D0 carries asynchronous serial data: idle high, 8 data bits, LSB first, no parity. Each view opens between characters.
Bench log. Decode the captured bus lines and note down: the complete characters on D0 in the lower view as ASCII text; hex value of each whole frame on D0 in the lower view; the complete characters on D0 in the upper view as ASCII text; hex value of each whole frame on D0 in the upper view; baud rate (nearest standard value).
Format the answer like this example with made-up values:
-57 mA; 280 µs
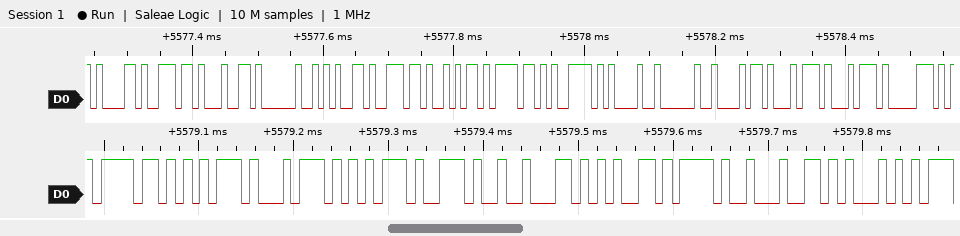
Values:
"outu.be/dQ"; 6F, 75, 74, 75, 2E, 62, 65, 2F, 64, 51; "and enjoy! http"; 61, 6E, 64, 20, 65, 6E, 6A, 6F, 79, 21, 20, 68, 74, 74, 70; 115200 baud
